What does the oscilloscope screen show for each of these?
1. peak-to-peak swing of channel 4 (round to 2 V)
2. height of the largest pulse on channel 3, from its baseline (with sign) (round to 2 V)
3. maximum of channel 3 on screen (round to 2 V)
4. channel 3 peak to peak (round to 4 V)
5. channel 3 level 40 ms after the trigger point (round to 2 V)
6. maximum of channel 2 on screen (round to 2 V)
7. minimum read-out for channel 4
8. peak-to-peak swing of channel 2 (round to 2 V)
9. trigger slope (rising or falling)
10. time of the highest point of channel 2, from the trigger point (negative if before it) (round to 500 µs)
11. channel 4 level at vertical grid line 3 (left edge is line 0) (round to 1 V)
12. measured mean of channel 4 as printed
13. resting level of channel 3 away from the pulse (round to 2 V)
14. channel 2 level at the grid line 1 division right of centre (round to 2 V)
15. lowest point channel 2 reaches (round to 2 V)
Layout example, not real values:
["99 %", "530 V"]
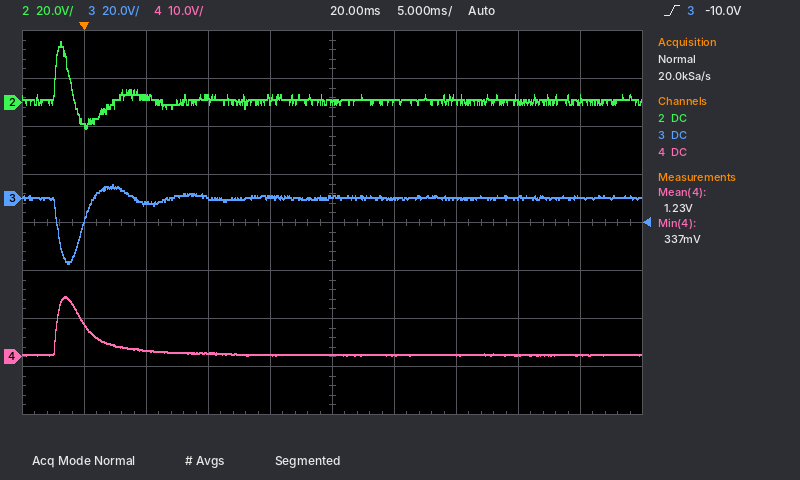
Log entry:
["12 V", "-28 V", "6 V", "32 V", "0 V", "26 V", "337 mV", "36 V", "rising", "-2.0 ms", "1 V", "1.23 V", "0 V", "0 V", "-10 V"]
